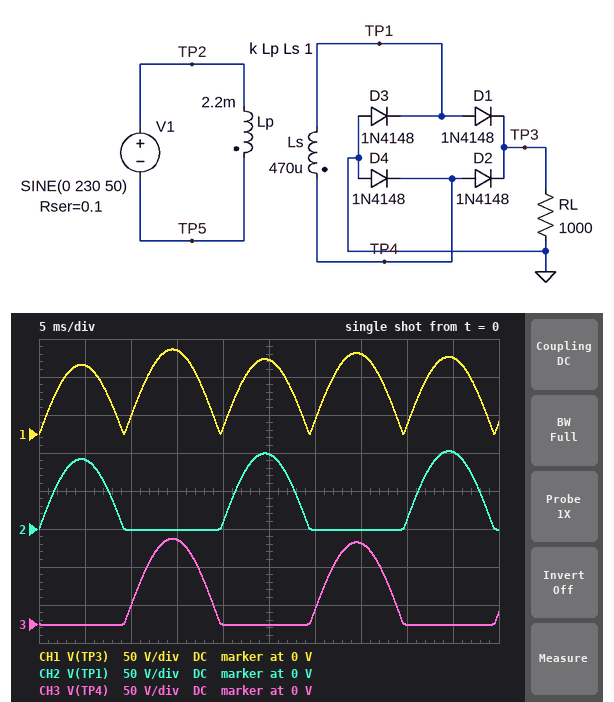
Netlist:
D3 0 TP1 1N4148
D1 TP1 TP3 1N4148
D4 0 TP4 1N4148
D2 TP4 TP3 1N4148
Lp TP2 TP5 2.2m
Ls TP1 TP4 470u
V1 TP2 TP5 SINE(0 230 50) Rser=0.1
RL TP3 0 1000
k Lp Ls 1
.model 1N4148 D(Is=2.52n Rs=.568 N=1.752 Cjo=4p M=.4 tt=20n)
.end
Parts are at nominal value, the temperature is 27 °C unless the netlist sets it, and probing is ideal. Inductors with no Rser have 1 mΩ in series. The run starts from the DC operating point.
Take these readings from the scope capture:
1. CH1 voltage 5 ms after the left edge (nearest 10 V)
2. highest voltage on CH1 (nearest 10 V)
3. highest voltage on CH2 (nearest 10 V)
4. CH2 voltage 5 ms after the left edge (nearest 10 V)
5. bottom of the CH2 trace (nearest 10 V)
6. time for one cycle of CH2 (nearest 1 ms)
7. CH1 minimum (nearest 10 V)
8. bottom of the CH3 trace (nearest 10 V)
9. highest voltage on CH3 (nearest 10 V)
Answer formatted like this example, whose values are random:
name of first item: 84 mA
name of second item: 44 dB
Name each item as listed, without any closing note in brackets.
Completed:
CH1 voltage 5 ms after the left edge: 90 V
highest voltage on CH1: 110 V
highest voltage on CH2: 100 V
CH2 voltage 5 ms after the left edge: 90 V
bottom of the CH2 trace: 0 V
time for one cycle of CH2: 20 ms
CH1 minimum: 0 V
bottom of the CH3 trace: 0 V
highest voltage on CH3: 110 V
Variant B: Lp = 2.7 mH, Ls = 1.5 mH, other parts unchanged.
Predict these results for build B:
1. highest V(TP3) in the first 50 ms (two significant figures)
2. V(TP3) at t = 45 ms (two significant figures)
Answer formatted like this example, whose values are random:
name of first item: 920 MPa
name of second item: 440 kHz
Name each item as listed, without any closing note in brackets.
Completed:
highest V(TP3) in the first 50 ms: 180 V
V(TP3) at t = 45 ms: 160 V
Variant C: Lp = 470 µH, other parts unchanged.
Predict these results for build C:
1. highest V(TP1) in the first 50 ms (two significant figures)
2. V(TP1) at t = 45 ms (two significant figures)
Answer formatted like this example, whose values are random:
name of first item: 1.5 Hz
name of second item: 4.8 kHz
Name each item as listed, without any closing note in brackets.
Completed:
highest V(TP1) in the first 50 ms: 190 V
V(TP1) at t = 45 ms: 160 V
